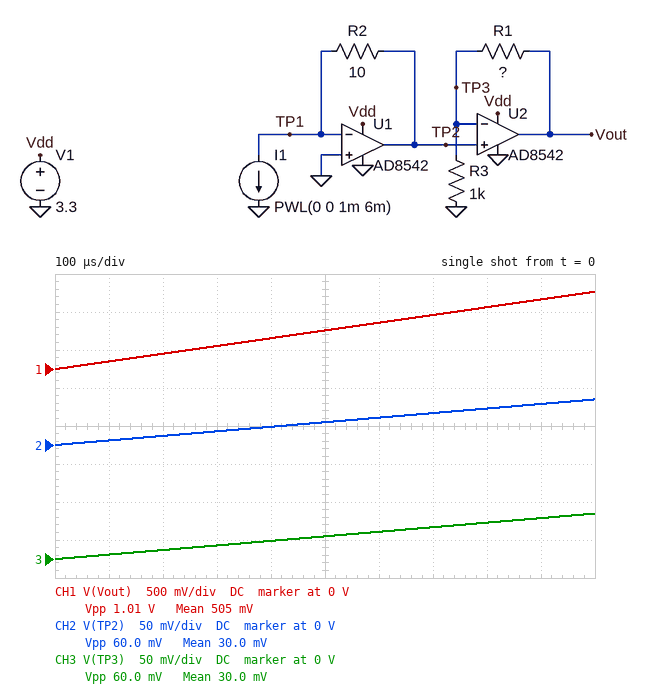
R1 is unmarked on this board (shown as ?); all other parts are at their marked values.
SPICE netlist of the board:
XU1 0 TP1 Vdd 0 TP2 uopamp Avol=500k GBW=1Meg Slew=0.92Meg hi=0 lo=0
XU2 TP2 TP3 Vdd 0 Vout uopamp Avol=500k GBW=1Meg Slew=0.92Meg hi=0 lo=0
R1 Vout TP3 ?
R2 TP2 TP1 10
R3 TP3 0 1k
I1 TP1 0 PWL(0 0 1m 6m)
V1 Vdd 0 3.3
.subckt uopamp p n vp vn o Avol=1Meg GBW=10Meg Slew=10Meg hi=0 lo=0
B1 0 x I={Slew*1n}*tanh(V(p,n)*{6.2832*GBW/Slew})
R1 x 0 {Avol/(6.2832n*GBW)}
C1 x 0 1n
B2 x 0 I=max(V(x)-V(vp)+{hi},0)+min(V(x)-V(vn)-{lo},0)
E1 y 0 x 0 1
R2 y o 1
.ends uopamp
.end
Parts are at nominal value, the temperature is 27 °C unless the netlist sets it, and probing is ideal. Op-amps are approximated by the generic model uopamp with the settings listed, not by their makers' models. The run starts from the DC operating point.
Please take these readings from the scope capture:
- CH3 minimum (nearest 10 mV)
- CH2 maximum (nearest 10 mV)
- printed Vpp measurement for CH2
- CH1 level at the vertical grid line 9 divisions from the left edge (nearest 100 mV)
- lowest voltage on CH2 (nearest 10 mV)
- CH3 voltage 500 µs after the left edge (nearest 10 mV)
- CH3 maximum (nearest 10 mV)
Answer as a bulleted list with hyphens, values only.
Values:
- 0 V
- 60 mV
- 60.0 mV
- 900 mV
- 0 V
- 30 mV
- 60 mV
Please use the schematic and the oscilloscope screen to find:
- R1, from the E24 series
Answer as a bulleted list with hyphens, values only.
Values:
- 16 kΩ
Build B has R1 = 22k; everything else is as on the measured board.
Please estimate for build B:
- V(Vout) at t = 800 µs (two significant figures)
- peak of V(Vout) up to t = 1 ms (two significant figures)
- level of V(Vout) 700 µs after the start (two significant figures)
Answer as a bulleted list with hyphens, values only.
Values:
- 1.1 V
- 1.4 V
- 960 mV
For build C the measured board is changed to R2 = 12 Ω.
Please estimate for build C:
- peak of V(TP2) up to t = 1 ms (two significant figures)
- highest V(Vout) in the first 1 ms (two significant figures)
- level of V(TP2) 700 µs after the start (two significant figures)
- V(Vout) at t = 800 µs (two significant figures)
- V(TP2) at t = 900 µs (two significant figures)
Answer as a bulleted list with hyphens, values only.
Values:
- 72 mV
- 1.2 V
- 50 mV
- 980 mV
- 65 mV
